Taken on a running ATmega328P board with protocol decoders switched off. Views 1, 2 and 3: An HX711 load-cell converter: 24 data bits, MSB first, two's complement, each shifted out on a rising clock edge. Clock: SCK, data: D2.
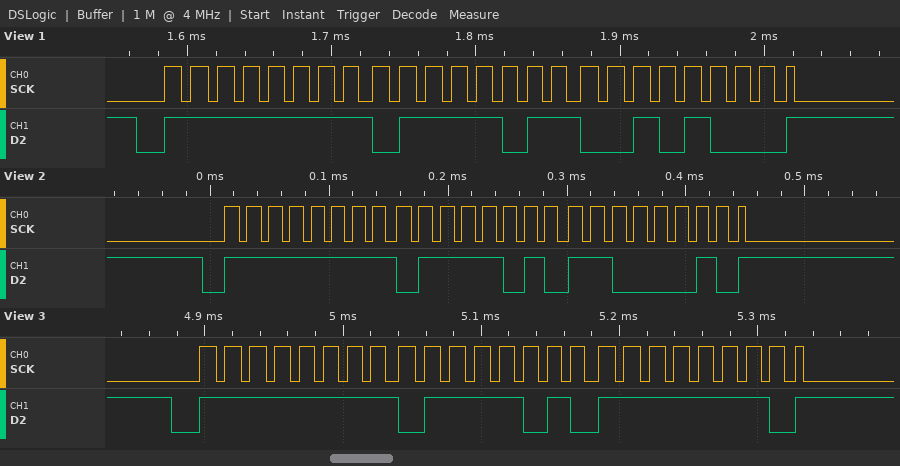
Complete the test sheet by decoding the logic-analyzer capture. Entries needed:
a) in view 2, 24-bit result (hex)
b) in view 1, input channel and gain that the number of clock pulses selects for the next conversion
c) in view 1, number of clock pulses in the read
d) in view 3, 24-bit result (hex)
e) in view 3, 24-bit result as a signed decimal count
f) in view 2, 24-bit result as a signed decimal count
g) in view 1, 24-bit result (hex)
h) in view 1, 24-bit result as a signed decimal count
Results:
0xFF7AC2
channel A, gain 128
25
0xFF7AFE
-34050
-34110
0xFF7B28
-34008
